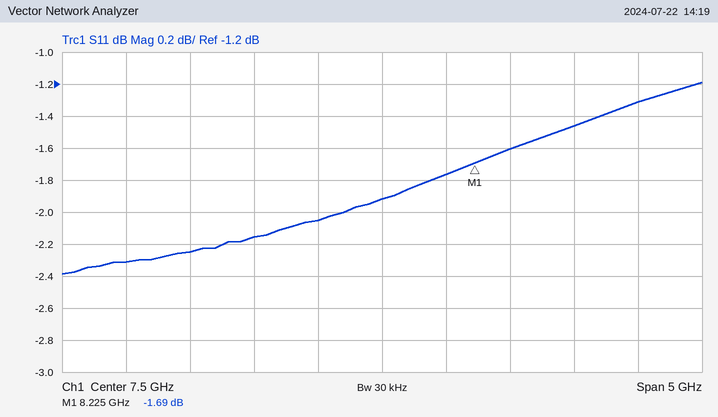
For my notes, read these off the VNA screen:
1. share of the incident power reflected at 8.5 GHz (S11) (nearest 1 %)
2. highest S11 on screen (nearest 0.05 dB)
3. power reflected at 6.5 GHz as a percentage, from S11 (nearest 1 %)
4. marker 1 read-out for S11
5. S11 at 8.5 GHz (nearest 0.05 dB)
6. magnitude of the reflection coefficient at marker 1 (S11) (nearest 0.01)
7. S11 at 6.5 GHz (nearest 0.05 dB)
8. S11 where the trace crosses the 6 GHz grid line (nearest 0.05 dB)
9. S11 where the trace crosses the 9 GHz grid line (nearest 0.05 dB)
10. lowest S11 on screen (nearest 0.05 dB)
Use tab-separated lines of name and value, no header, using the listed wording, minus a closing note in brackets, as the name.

share of the incident power reflected at 8.5 GHz (S11)	69 %
highest S11 on screen	-1.20 dB
power reflected at 6.5 GHz as a percentage, from S11	61 %
marker 1 read-out for S11	-1.69 dB
S11 at 8.5 GHz	-1.60 dB
magnitude of the reflection coefficient at marker 1 (S11)	0.82
S11 at 6.5 GHz	-2.15 dB
S11 where the trace crosses the 6 GHz grid line	-2.25 dB
S11 where the trace crosses the 9 GHz grid line	-1.45 dB
lowest S11 on screen	-2.40 dB
